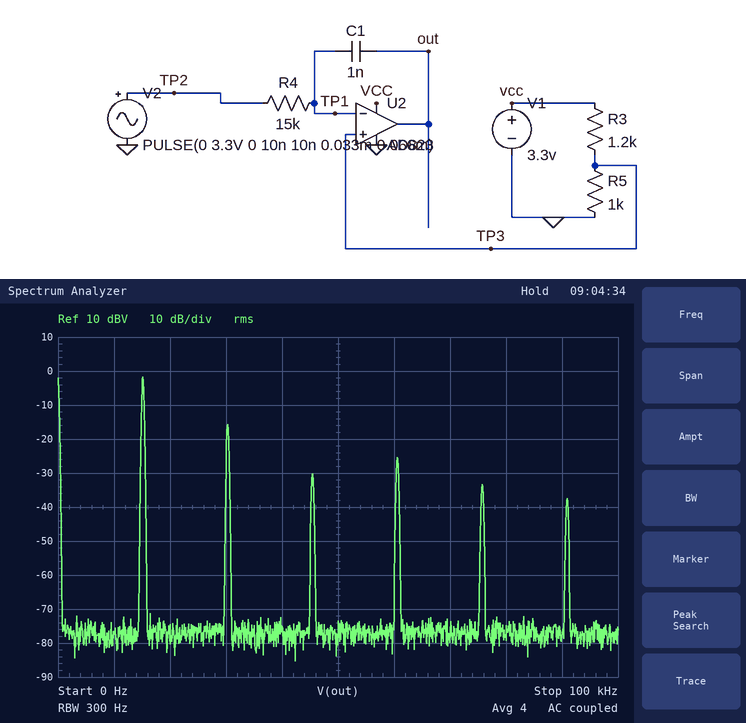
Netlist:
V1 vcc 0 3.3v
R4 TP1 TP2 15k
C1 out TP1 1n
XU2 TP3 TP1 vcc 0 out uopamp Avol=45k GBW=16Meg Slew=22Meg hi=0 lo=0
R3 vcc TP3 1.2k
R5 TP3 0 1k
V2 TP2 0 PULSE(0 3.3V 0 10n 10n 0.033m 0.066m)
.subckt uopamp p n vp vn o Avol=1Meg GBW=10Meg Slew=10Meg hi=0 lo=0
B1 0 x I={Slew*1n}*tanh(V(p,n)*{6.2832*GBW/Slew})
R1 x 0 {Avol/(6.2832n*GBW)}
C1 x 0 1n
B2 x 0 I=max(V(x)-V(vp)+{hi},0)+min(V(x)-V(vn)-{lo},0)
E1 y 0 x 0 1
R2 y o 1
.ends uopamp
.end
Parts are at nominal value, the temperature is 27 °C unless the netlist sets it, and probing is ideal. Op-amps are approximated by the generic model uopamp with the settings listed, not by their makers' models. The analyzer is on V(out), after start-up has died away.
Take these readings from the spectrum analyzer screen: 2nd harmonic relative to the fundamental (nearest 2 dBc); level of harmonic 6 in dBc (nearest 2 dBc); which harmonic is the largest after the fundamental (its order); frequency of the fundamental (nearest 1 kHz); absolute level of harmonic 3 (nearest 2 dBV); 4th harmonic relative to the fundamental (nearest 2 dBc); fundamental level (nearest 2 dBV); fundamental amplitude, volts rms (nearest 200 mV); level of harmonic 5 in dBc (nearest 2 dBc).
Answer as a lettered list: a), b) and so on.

a) -14 dBc
b) -36 dBc
c) 2
d) 15 kHz
e) -30 dBV
f) -24 dBc
g) -2 dBV
h) 800 mV
i) -32 dBc
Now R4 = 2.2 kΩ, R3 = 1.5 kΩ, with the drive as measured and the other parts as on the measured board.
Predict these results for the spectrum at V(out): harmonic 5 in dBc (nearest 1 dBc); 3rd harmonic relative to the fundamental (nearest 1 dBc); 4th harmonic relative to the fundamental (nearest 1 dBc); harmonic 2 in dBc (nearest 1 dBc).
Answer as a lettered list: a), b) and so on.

a) -17 dBc
b) -10 dBc
c) -22 dBc
d) -21 dBc
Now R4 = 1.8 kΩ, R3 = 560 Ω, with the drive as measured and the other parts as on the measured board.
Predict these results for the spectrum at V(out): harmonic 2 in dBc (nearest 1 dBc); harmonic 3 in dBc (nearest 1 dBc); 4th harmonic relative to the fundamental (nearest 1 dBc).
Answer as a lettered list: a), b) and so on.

a) -20 dBc
b) -10 dBc
c) -21 dBc
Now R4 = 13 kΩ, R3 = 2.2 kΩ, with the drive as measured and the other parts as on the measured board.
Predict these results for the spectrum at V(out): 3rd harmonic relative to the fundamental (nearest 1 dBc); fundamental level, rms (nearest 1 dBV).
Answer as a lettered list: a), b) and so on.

a) -12 dBc
b) -8 dBV
